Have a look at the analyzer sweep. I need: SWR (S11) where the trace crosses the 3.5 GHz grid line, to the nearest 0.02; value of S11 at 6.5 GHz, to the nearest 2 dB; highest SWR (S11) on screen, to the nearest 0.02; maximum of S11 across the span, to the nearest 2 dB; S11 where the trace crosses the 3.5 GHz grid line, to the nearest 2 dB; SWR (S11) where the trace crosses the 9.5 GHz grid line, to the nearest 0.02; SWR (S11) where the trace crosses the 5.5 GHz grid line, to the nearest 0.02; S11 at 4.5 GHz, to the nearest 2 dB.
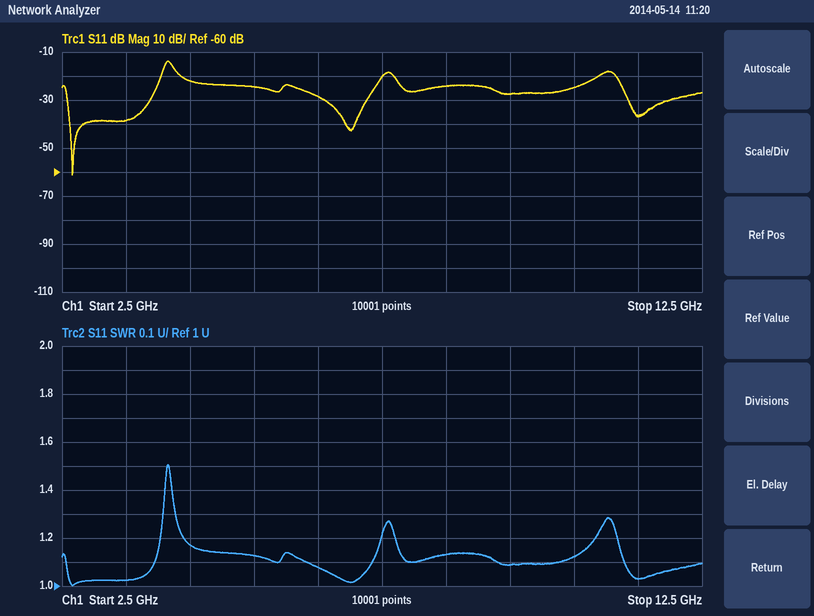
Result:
1.02
-28 dB
1.50
-14 dB
-38 dB
1.08
1.12
-22 dB
